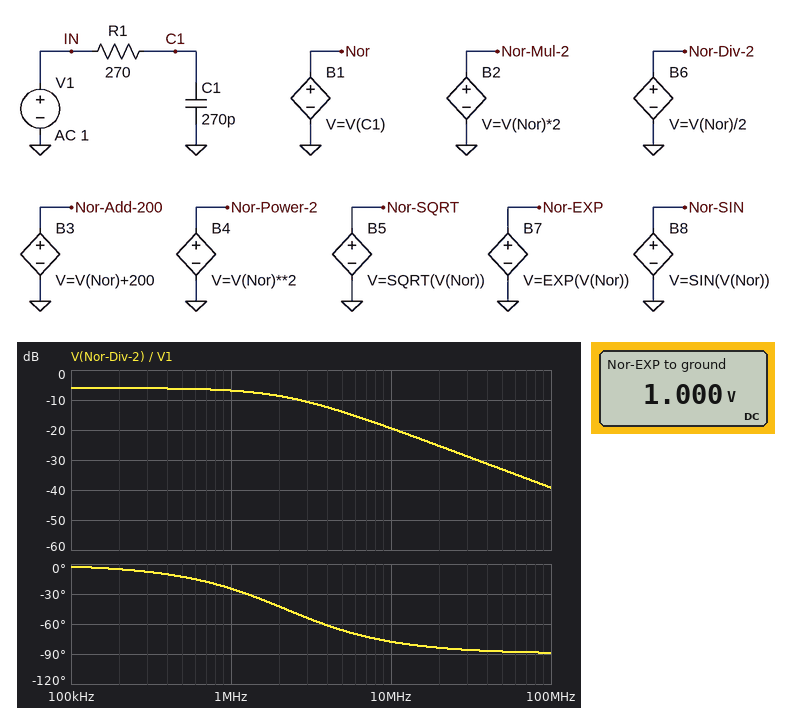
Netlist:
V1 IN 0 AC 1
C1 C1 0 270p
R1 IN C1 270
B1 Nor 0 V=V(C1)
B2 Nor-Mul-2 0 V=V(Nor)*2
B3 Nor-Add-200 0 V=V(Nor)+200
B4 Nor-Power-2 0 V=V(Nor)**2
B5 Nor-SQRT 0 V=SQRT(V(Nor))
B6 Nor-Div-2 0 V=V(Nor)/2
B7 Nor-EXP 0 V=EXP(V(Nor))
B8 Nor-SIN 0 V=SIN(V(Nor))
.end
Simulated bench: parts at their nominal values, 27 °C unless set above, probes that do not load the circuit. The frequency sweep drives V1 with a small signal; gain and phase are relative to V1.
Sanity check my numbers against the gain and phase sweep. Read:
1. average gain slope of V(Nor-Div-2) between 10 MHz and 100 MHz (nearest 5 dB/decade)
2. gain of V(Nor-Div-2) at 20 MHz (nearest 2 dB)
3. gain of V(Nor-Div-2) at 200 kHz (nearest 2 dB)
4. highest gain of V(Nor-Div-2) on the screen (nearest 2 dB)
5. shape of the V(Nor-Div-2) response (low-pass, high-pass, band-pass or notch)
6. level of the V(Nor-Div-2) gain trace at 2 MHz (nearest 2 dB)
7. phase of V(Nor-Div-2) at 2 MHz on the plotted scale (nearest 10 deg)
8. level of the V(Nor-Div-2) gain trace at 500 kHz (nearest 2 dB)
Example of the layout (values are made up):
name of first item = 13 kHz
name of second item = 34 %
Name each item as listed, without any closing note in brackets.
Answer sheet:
average gain slope of V(Nor-Div-2) between 10 MHz and 100 MHz = -20 dB/decade
gain of V(Nor-Div-2) at 20 MHz = -26 dB
gain of V(Nor-Div-2) at 200 kHz = -6 dB
highest gain of V(Nor-Div-2) on the screen = -6 dB
shape of the V(Nor-Div-2) response = low-pass
level of the V(Nor-Div-2) gain trace at 2 MHz = -8 dB
phase of V(Nor-Div-2) at 2 MHz on the plotted scale = -40 deg
level of the V(Nor-Div-2) gain trace at 500 kHz = -6 dB
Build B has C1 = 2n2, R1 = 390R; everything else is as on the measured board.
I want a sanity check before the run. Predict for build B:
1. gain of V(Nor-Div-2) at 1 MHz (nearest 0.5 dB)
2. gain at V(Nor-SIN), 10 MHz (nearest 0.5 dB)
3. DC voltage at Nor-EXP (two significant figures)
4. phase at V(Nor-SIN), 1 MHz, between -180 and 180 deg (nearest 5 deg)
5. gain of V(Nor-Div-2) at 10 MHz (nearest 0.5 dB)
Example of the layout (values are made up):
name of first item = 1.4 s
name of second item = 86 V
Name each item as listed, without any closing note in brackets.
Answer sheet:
gain of V(Nor-Div-2) at 1 MHz = -21.0 dB
gain at V(Nor-SIN), 10 MHz = -34.5 dB
DC voltage at Nor-EXP = 1.0 V
phase at V(Nor-SIN), 1 MHz, between -180 and 180 deg = -80 deg
gain of V(Nor-Div-2) at 10 MHz = -40.5 dB
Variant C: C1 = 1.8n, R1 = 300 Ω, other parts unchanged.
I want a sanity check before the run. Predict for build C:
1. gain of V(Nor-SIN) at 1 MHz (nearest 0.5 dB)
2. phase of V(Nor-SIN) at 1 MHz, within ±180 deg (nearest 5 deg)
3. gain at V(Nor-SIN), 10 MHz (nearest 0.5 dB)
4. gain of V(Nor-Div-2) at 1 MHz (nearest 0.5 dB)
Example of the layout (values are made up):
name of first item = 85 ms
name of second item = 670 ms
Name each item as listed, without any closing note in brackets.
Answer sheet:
gain of V(Nor-SIN) at 1 MHz = -11.0 dB
phase of V(Nor-SIN) at 1 MHz, within ±180 deg = -75 deg
gain at V(Nor-SIN), 10 MHz = -30.5 dB
gain of V(Nor-Div-2) at 1 MHz = -17.0 dB
